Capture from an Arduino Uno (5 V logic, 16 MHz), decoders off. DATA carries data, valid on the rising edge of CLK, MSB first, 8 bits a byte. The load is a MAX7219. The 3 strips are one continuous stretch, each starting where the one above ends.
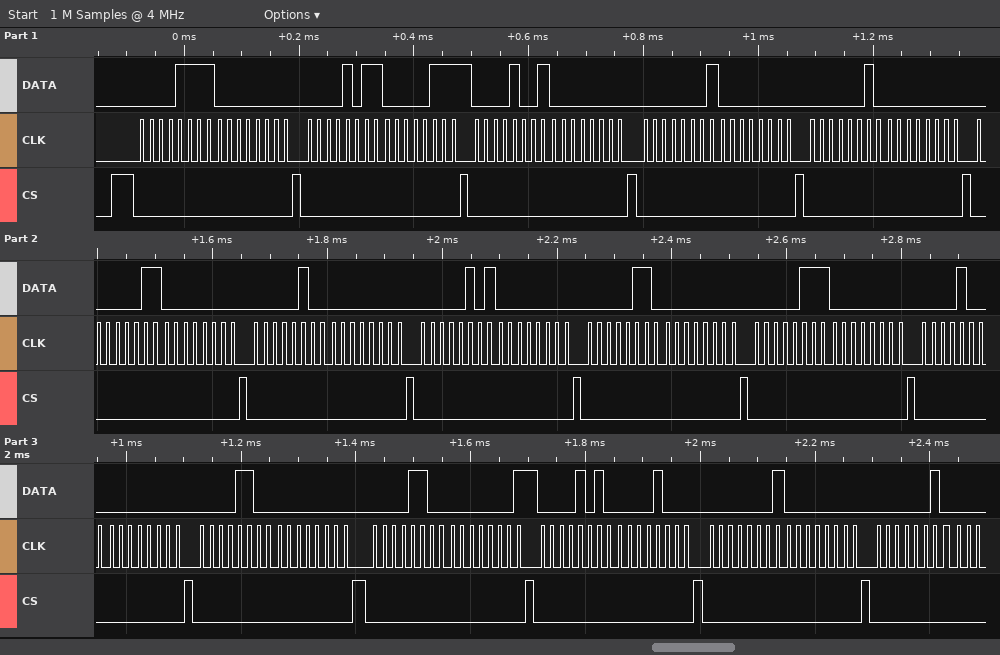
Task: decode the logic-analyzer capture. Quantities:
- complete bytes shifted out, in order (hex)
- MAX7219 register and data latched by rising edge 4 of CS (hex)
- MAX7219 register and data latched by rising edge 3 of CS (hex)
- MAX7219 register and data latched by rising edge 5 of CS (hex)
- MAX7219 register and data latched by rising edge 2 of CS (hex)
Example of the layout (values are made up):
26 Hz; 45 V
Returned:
0F 00 0B 07 09 00 01 00 02 00 03 00 04 00 05 00 06 00 07 00 08 00 0C 00 0C 01 0A 08 01 00 02; register 0x9, data 0x00; register 0xB, data 0x07; register 0x1, data 0x00; register 0xF, data 0x00
